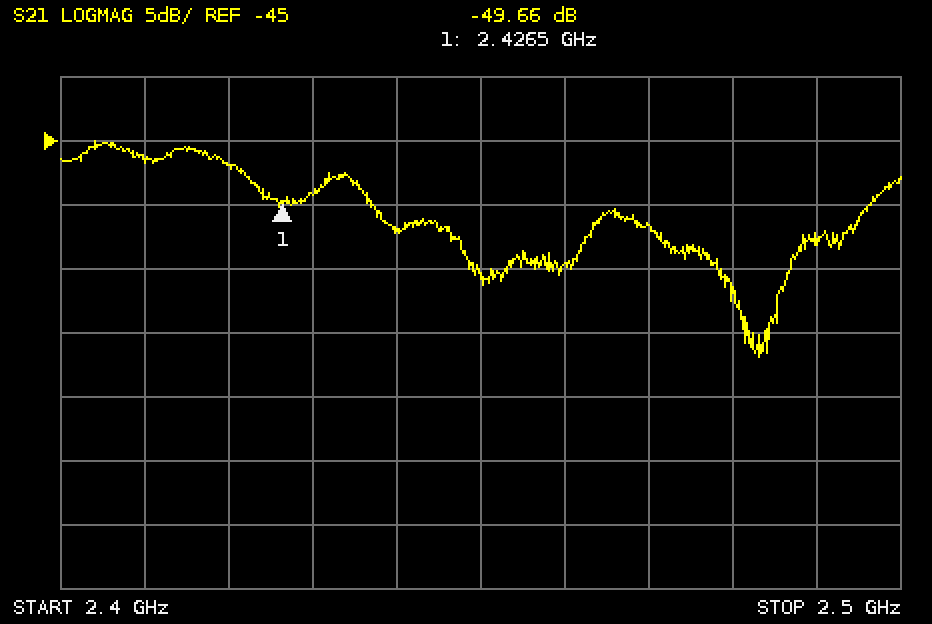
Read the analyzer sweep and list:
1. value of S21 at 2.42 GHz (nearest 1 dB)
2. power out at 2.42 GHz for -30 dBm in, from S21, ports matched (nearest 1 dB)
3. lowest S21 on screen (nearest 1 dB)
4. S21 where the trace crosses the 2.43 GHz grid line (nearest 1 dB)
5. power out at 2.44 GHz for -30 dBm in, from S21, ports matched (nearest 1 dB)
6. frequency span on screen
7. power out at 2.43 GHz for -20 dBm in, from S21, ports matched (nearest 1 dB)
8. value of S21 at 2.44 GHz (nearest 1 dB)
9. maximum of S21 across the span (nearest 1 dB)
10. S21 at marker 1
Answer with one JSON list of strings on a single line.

["-47 dB", "-77 dBm", "-62 dB", "-49 dB", "-82 dBm", "100 MHz", "-69 dBm", "-52 dB", "-45 dB", "-49.66 dB"]
